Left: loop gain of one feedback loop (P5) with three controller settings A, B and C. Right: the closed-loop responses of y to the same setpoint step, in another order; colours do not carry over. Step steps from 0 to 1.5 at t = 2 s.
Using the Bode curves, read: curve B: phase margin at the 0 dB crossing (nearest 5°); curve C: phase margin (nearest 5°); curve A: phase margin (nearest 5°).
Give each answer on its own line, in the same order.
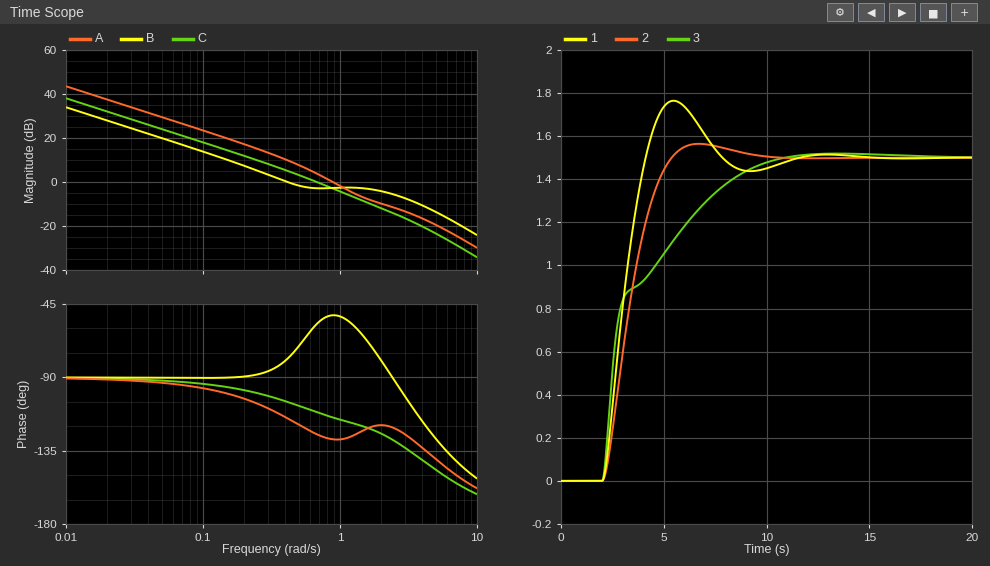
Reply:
100°
70°
50°
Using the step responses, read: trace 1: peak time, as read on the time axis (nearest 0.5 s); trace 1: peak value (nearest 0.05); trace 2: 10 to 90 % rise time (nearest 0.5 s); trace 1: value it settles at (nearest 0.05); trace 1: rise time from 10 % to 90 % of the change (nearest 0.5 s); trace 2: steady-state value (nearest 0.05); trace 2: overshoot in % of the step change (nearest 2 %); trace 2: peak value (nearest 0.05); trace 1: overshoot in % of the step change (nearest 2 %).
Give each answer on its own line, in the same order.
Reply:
5.5 s
1.75
2.0 s
1.50
1.5 s
1.50
4 %
1.55
18 %
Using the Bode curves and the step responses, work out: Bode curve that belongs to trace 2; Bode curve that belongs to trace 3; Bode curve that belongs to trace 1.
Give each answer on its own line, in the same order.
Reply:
C
B
A
